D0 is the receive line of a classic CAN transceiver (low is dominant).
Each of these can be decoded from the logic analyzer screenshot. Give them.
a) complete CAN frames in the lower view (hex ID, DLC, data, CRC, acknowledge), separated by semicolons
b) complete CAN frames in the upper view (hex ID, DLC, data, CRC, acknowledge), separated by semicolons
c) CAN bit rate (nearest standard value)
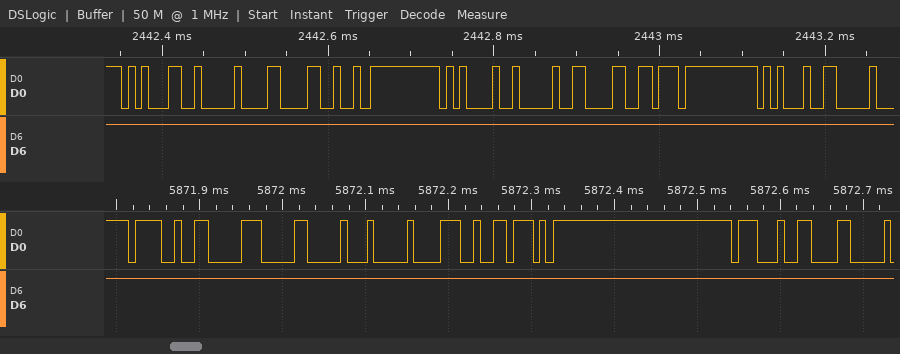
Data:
ID 793, DLC 3, data 04 02 00, CRC 726E, ACK
ID 519, DLC 0, CRC 1864, ACK; ID 509, DLC 0, CRC 619B, ACK
125 kbit/s
